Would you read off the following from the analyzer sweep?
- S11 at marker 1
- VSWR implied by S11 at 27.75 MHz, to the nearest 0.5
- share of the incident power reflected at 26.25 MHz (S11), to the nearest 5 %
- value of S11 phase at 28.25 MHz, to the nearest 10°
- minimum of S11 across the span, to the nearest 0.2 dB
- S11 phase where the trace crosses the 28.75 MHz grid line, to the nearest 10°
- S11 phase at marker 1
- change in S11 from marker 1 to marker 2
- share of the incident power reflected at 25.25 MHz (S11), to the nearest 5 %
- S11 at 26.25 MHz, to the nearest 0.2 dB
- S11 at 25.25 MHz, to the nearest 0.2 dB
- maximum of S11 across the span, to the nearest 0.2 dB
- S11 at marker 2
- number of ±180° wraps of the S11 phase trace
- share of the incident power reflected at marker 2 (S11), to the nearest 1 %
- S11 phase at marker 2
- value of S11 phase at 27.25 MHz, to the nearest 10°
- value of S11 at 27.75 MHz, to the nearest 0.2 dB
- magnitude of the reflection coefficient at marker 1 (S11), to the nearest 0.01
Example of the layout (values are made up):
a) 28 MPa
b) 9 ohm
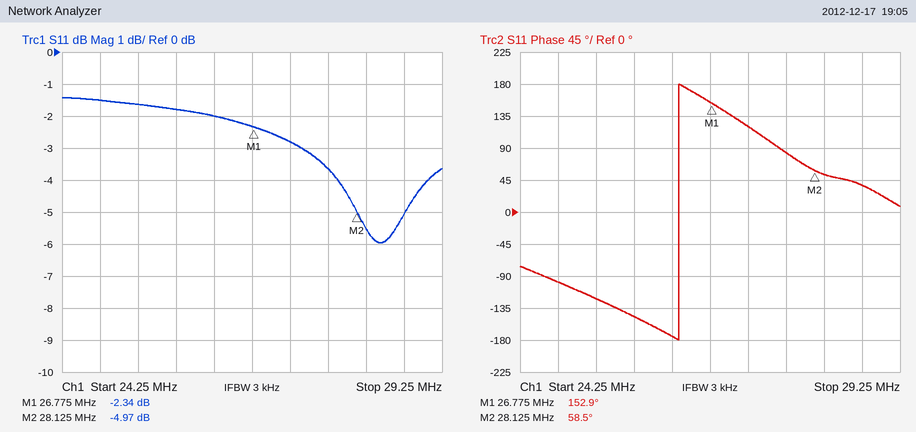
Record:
a) -2.34 dB
b) 5.0
c) 65 %
d) 50°
e) -6.0 dB
f) 40°
g) 152.9°
h) -2.63 dB
i) 70 %
j) -2.0 dB
k) -1.6 dB
l) -1.4 dB
m) -4.97 dB
n) 1
o) 32 %
p) 58.5°
q) 120°
r) -3.6 dB
s) 0.76
